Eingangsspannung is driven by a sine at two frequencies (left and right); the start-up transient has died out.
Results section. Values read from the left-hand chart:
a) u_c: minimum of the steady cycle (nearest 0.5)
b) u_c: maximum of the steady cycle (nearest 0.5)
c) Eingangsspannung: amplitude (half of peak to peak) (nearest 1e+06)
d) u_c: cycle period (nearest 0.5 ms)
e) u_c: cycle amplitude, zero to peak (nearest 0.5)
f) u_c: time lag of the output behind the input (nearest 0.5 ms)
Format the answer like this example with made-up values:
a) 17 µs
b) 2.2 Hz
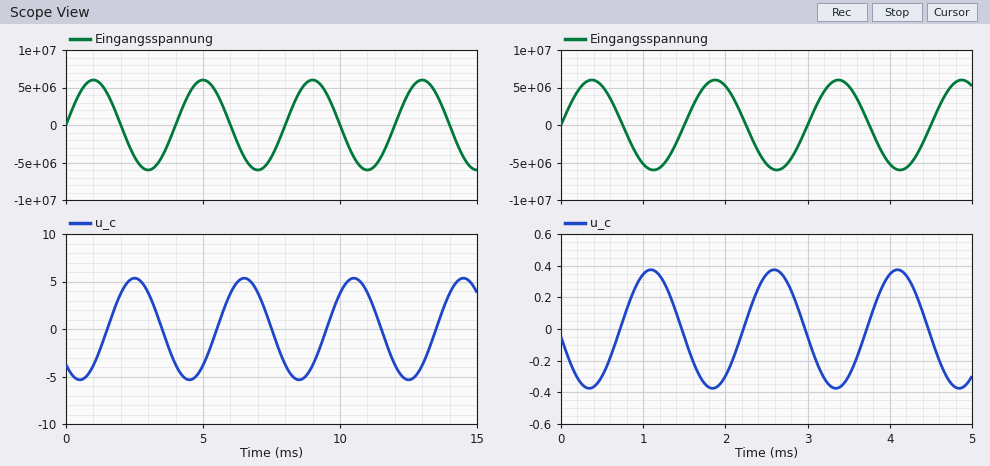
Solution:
a) -5.5
b) 5.5
c) 6000000
d) 4.0 ms
e) 5.5
f) 1.5 ms
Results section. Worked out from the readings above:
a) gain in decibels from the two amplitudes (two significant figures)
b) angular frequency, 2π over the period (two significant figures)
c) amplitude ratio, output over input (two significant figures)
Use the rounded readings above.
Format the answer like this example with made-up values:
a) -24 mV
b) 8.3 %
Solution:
a) -120 dB
b) 1.6 rad/ms
c) 0.00000092
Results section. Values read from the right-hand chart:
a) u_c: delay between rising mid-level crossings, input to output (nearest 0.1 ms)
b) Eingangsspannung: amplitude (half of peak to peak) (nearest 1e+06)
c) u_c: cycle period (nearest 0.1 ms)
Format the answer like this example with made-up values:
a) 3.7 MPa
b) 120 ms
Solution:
a) 0.7 ms
b) 6000000
c) 1.5 ms
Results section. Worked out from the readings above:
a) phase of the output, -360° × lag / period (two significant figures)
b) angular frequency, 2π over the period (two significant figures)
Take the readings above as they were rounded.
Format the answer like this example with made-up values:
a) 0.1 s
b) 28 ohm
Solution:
a) -170°
b) 4.2 rad/ms
